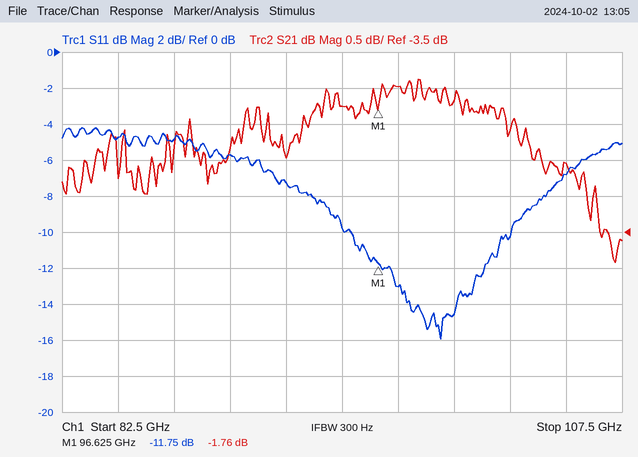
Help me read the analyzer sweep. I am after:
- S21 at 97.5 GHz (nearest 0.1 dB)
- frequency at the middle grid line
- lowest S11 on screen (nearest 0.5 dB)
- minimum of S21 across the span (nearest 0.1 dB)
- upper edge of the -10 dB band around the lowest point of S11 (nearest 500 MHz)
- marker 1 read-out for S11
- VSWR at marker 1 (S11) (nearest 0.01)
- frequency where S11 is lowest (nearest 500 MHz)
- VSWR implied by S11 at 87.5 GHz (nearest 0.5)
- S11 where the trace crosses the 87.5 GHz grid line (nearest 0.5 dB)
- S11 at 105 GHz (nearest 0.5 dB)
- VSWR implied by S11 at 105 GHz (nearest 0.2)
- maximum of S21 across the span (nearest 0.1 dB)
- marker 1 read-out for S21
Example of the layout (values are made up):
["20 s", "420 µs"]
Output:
["-1.5 dB", "95 GHz", "-16.0 dB", "-3.9 dB", "102.5 GHz", "-11.75 dB", "1.70", "99.5 GHz", "3.5", "-5.0 dB", "-7.0 dB", "2.6", "-1.4 dB", "-1.76 dB"]
